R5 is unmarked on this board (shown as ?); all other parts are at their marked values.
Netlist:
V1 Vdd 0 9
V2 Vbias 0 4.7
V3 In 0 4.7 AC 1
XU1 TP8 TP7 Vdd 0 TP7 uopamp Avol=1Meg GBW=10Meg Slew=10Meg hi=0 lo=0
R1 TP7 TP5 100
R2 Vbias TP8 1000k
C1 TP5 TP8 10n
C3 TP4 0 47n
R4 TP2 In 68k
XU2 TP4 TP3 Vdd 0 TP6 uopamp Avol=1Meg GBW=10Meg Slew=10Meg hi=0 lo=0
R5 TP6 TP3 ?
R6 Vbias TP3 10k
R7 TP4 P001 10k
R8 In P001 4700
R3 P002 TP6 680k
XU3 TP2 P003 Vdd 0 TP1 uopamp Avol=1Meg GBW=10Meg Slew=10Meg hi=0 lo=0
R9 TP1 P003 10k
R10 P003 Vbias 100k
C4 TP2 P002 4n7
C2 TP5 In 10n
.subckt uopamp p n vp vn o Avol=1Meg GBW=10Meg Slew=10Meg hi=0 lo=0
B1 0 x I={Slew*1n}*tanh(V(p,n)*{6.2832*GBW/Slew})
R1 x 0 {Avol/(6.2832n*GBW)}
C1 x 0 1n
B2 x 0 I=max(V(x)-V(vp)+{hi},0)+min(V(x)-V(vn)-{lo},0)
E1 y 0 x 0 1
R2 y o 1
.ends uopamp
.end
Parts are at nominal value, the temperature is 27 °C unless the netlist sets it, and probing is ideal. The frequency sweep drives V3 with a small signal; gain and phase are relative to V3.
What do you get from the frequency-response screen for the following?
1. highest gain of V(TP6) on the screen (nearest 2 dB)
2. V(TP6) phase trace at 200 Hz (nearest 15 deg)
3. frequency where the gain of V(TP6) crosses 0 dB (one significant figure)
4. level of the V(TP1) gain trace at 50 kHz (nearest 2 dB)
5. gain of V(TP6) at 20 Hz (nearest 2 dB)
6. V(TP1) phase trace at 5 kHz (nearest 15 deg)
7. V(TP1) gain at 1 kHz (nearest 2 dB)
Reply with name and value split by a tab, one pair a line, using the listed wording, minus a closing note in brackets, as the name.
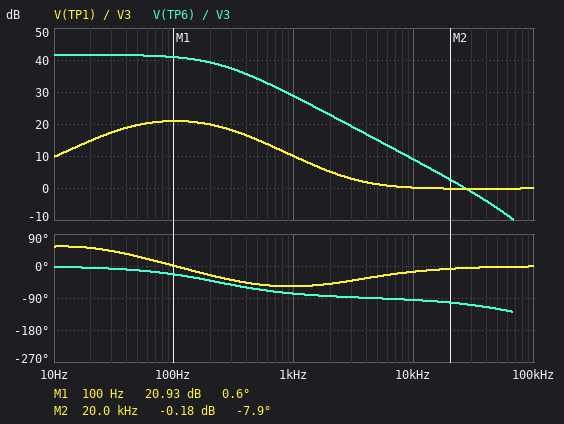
highest gain of V(TP6) on the screen	42 dB
V(TP6) phase trace at 200 Hz	-45 deg
frequency where the gain of V(TP6) crosses 0 dB	30 kHz
level of the V(TP1) gain trace at 50 kHz	0 dB
gain of V(TP6) at 20 Hz	42 dB
V(TP1) phase trace at 5 kHz	-30 deg
V(TP1) gain at 1 kHz	10 dB
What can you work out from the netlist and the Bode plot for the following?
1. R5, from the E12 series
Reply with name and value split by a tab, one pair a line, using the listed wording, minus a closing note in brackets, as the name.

R5, from the E12 series	1.2 MΩ
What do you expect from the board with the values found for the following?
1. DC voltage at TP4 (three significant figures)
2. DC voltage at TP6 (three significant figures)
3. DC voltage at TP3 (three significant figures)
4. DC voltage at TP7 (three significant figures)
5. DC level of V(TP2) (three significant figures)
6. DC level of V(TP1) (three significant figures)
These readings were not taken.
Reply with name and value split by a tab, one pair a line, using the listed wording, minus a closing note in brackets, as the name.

DC voltage at TP4	4.70 V
DC voltage at TP6	4.70 V
DC voltage at TP3	4.70 V
DC voltage at TP7	4.70 V
DC level of V(TP2)	4.70 V
DC level of V(TP1)	4.70 V
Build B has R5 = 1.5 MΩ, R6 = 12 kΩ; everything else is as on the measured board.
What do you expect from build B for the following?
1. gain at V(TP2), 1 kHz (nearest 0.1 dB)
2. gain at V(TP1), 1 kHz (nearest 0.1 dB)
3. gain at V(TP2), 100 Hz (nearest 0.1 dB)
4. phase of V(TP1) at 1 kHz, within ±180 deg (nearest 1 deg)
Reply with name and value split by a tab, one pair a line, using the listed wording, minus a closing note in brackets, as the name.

gain at V(TP2), 1 kHz	9.4 dB
gain at V(TP1), 1 kHz	10.2 dB
gain at V(TP2), 100 Hz	20.4 dB
phase of V(TP1) at 1 kHz, within ±180 deg	-58 deg
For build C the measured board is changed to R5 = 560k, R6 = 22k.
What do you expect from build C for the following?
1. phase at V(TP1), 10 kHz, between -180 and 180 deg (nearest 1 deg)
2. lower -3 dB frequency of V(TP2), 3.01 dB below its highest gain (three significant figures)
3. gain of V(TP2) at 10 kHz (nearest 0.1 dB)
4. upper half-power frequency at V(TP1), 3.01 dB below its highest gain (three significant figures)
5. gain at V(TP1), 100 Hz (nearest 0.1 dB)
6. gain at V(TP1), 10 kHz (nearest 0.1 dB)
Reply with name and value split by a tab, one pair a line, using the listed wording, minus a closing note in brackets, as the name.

phase at V(TP1), 10 kHz, between -180 and 180 deg	-4 deg
lower -3 dB frequency of V(TP2), 3.01 dB below its highest gain	30.2 Hz
gain of V(TP2) at 10 kHz	-0.8 dB
upper half-power frequency at V(TP1), 3.01 dB below its highest gain	337 Hz
gain at V(TP1), 100 Hz	10.2 dB
gain at V(TP1), 10 kHz	0 dB
